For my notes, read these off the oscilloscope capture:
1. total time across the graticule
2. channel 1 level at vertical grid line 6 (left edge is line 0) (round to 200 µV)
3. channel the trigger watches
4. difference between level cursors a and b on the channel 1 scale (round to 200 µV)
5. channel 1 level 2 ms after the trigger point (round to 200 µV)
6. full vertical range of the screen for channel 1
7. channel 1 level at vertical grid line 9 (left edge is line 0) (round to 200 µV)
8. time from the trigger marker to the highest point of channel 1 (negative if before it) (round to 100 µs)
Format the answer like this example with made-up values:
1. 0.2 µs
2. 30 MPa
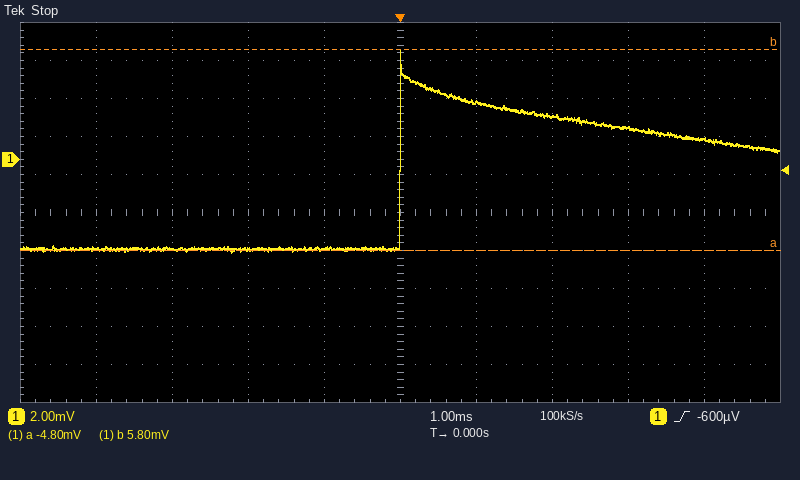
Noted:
1. 10 ms
2. 3.0 mV
3. channel 1
4. 10.6 mV
5. 2.2 mV
6. 20 mV
7. 1.0 mV
8. 0.0 ms
